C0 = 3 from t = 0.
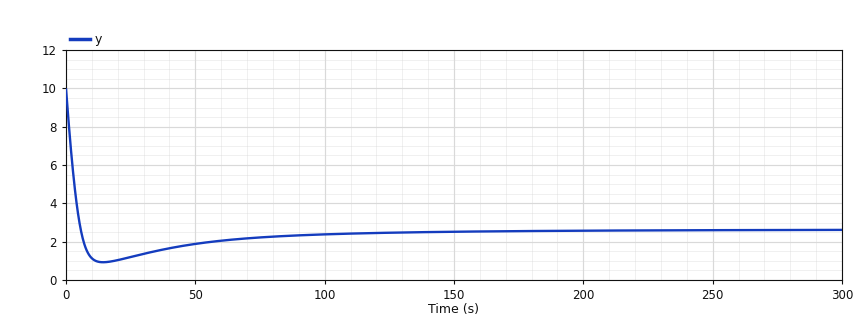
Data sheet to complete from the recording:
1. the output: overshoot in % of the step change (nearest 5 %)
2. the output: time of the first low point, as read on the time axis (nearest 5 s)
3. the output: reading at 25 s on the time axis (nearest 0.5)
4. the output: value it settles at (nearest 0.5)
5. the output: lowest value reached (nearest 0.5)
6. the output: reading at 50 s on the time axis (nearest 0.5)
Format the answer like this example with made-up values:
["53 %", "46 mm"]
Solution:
["25 %", "15 s", "1.0", "2.5", "1.0", "2.0"]
